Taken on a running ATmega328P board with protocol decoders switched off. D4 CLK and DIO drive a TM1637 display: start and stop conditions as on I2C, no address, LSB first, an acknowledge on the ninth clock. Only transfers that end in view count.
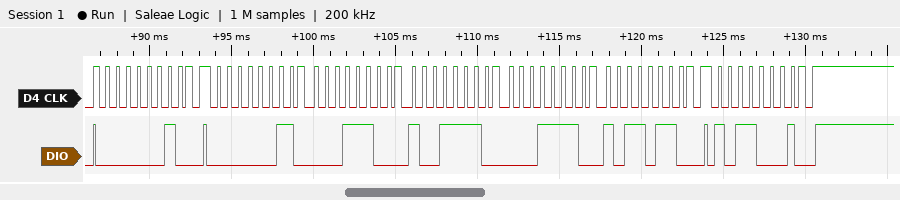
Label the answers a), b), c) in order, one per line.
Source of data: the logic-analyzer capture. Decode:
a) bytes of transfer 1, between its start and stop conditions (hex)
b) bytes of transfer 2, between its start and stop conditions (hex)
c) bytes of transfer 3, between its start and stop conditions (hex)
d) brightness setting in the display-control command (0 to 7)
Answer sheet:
a) 40
b) C0 38 79 78 6D
c) 8D
d) 5
